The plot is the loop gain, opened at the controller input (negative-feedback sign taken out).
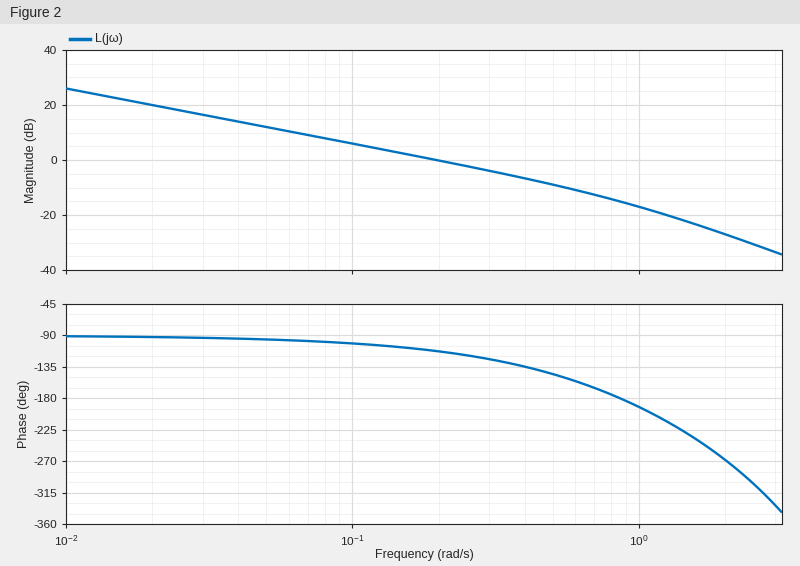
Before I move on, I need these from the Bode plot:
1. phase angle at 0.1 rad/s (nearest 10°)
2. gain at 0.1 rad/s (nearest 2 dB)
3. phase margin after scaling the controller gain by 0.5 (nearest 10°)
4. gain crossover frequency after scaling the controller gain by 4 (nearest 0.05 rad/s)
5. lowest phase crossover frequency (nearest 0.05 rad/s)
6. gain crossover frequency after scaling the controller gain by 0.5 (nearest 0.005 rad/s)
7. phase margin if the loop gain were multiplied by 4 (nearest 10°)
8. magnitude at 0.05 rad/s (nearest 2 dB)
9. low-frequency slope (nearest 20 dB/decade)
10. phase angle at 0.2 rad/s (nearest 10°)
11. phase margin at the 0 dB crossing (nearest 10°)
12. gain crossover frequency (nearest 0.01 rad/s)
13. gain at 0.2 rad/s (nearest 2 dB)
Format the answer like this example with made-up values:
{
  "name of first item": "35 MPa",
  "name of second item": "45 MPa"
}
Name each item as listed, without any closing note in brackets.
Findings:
{
  "phase angle at 0.1 rad/s": "-100°",
  "gain at 0.1 rad/s": "6 dB",
  "phase margin after scaling the controller gain by 0.5": "80°",
  "gain crossover frequency after scaling the controller gain by 4": "0.65 rad/s",
  "lowest phase crossover frequency": "0.85 rad/s",
  "gain crossover frequency after scaling the controller gain by 0.5": "0.100 rad/s",
  "phase margin if the loop gain were multiplied by 4": "20°",
  "magnitude at 0.05 rad/s": "12 dB",
  "low-frequency slope": "-20 dB/decade",
  "phase angle at 0.2 rad/s": "-110°",
  "phase margin at the 0 dB crossing": "70°",
  "gain crossover frequency": "0.20 rad/s",
  "gain at 0.2 rad/s": "0 dB"
}
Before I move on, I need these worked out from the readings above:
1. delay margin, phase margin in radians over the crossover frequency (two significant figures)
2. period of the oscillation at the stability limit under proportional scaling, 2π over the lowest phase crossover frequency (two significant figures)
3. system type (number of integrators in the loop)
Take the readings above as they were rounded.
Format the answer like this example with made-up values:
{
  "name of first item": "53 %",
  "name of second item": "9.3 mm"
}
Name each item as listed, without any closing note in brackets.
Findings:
{
  "delay margin, phase margin in radians over the crossover frequency": "6.1 s",
  "period of the oscillation at the stability limit under proportional scaling, 2π over the lowest phase crossover frequency": "7.4 s",
  "system type": "1"
}
